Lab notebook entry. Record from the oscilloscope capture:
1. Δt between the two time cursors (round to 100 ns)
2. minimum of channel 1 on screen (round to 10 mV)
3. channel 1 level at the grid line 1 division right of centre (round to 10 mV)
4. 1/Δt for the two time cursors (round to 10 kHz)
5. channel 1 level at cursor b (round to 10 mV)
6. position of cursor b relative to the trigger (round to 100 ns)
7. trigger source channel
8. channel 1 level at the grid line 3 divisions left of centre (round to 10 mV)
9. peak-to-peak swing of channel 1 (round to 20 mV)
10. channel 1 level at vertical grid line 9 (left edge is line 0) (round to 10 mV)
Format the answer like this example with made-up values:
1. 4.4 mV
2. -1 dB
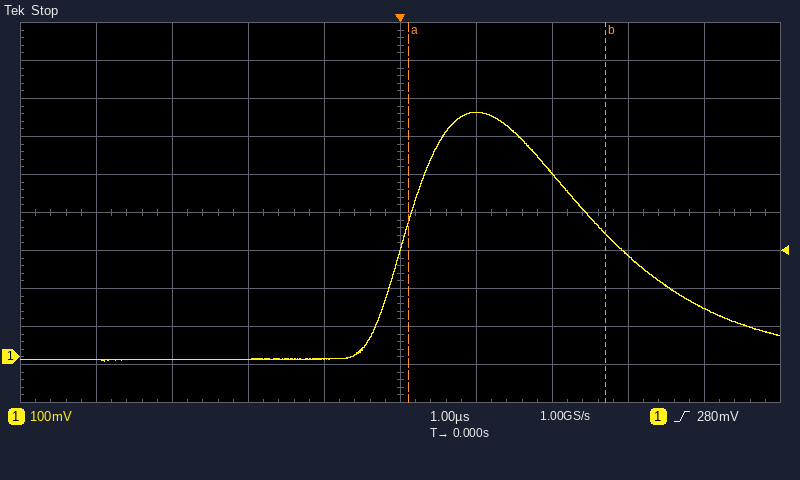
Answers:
1. 2.6 µs
2. -10 mV
3. 640 mV
4. 380 kHz
5. 320 mV
6. +2.7 µs
7. channel 1
8. -10 mV
9. 660 mV
10. 130 mV
